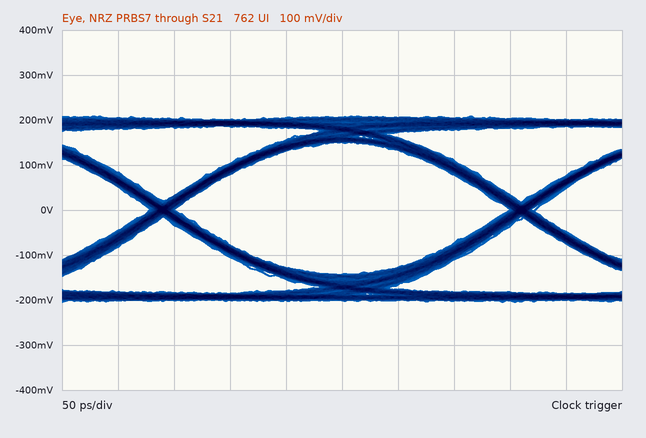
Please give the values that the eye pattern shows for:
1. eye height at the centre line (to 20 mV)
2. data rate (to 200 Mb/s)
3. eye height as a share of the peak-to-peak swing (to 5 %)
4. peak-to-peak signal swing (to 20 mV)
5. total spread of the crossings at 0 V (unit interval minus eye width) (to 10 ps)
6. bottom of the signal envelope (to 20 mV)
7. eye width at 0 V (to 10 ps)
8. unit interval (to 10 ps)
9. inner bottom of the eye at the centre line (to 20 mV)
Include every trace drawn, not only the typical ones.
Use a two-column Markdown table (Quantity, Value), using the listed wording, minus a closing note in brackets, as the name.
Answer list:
| Quantity | Value |
|---|---|
| eye height at the centre line | 300 mV |
| data rate | 3.2 Gb/s |
| eye height as a share of the peak-to-peak swing | 70 % |
| peak-to-peak signal swing | 420 mV |
| total spread of the crossings at 0 V (unit interval minus eye width) | 20 ps |
| bottom of the signal envelope | -200 mV |
| eye width at 0 V | 300 ps |
| unit interval | 320 ps |
| inner bottom of the eye at the centre line | -140 mV |
